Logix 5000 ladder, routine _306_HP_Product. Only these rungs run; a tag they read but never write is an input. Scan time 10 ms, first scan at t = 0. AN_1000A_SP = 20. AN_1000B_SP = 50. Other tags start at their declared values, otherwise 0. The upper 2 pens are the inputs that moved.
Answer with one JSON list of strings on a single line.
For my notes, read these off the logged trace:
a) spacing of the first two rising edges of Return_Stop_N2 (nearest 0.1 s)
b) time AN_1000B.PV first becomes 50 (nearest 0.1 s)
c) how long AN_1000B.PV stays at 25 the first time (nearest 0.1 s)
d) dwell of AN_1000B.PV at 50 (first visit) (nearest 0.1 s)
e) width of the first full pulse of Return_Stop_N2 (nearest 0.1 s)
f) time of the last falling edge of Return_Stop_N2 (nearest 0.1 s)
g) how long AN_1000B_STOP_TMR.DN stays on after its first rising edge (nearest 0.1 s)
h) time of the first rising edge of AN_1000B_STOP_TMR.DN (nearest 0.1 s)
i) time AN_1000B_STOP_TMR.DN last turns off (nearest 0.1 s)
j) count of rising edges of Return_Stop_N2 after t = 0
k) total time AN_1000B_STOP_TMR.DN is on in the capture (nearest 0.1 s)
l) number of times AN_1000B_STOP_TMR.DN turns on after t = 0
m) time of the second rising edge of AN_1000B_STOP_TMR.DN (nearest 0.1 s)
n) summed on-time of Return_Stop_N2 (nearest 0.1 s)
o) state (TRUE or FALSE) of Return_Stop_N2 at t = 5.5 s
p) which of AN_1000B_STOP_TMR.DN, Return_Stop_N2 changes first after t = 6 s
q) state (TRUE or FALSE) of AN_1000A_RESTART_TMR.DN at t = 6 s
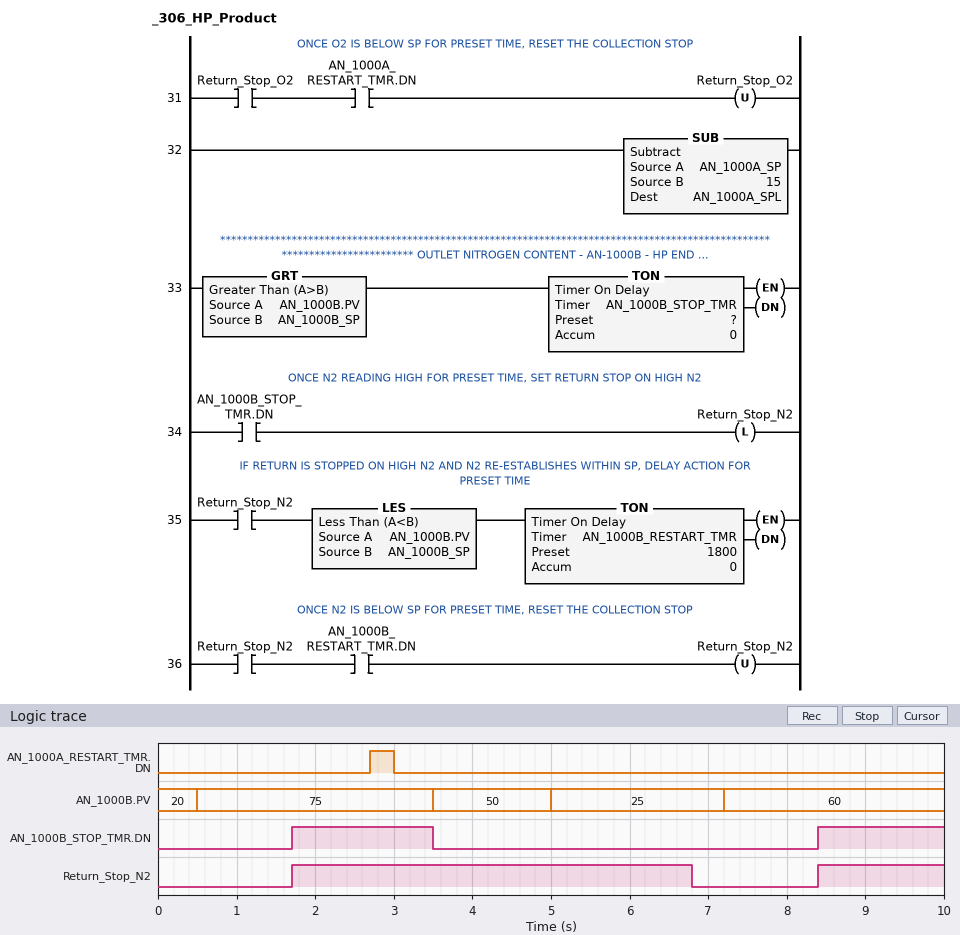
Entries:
["6.7 s", "3.5 s", "2.2 s", "1.5 s", "5.1 s", "6.8 s", "1.8 s", "1.7 s", "3.5 s", "2", "3.4 s", "2", "8.4 s", "6.7 s", "TRUE", "Return_Stop_N2", "FALSE"]
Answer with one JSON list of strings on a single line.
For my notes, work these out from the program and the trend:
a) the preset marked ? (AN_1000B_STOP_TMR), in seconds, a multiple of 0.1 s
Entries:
["1.2 s"]
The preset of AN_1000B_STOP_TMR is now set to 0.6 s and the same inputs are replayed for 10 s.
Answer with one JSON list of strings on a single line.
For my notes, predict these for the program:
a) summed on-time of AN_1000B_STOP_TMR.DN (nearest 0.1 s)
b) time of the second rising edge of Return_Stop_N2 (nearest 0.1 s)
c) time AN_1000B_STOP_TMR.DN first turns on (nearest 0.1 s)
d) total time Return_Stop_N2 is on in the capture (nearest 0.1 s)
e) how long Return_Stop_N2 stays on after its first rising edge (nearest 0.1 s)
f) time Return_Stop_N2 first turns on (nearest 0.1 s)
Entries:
["4.6 s", "7.8 s", "1.1 s", "7.9 s", "5.7 s", "1.1 s"]
